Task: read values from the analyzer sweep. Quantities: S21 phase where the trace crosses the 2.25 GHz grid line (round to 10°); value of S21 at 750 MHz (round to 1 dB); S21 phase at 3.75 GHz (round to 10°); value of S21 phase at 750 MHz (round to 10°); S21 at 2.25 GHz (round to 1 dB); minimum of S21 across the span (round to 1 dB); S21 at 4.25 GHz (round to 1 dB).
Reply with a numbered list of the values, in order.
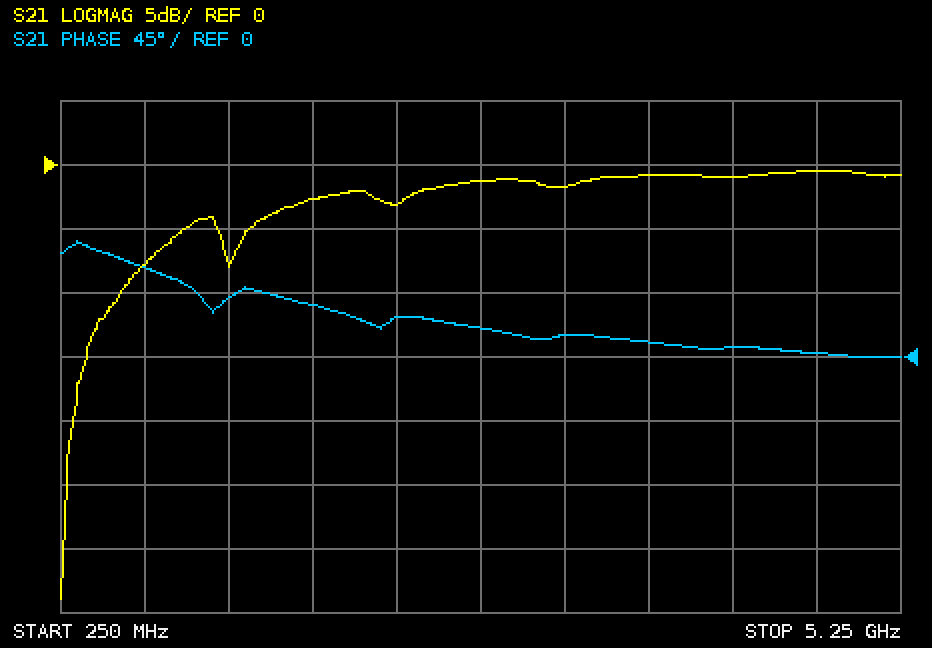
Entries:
1. 30°
2. -8 dB
3. 10°
4. 60°
5. -3 dB
6. -34 dB
7. -1 dB
